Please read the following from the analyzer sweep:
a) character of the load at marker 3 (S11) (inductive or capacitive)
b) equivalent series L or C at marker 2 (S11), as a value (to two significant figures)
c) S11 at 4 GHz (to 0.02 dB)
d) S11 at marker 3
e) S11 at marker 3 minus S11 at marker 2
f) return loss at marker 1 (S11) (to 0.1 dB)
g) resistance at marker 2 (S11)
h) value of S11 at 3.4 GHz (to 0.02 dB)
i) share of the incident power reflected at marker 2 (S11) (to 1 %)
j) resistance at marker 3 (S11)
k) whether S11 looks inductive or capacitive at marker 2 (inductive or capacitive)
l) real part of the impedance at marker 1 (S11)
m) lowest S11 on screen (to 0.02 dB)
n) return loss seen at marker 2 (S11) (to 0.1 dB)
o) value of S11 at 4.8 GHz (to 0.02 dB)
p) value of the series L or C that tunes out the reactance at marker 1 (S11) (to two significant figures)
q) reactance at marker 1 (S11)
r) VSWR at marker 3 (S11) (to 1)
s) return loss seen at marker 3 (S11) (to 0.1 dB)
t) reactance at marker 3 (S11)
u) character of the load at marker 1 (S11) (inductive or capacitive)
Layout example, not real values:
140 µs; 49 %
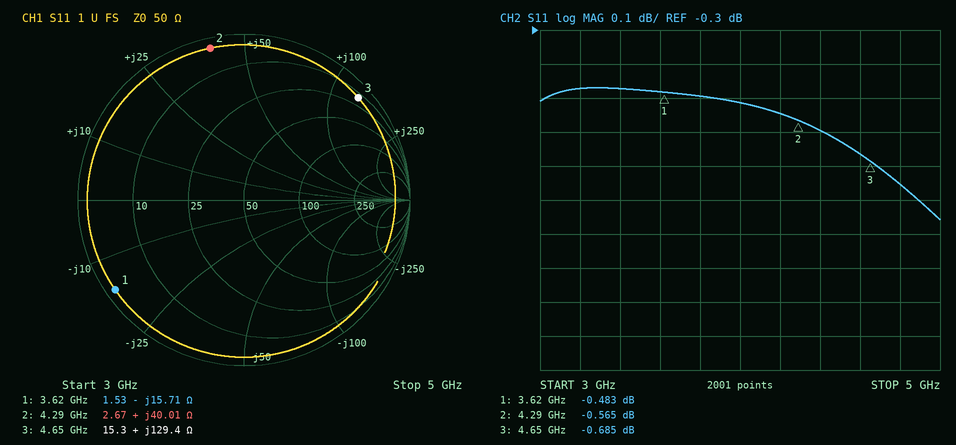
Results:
inductive; 1.5 nH; -0.52 dB; -0.685 dB; -0.120 dB; 0.5 dB; 2.67 Ω; -0.48 dB; 88 %; 15.3 Ω; inductive; 1.53 Ω; -0.86 dB; 0.6 dB; -0.76 dB; 690 pH; -15.71 Ω; 25; 0.7 dB; +129.4 Ω; capacitive
